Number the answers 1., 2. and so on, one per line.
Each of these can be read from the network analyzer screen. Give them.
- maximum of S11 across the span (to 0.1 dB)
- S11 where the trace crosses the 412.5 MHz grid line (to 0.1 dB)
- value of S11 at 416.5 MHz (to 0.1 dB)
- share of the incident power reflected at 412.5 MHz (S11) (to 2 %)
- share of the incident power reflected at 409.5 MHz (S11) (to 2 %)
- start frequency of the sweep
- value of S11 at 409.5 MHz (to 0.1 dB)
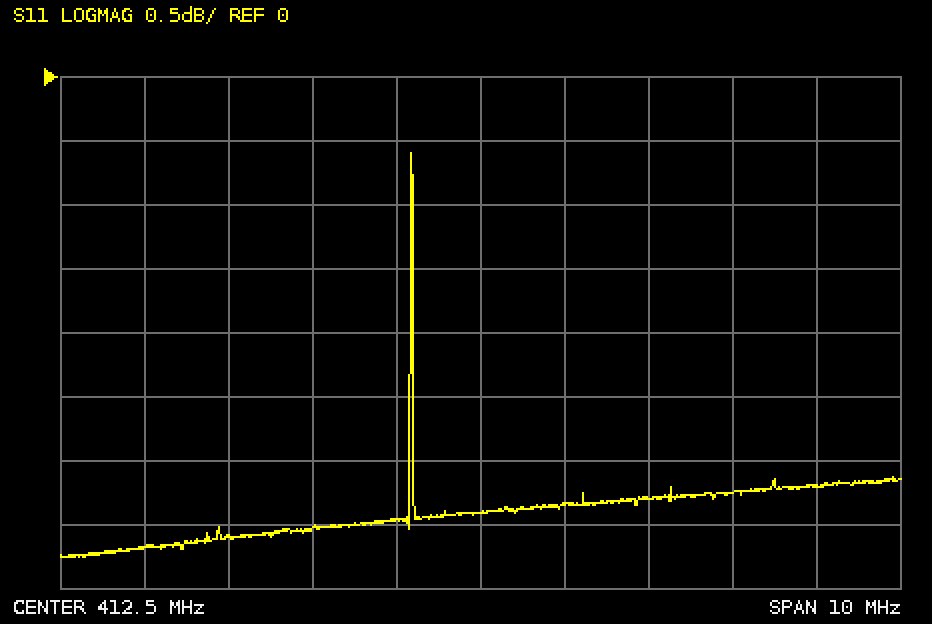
1. -0.6 dB
2. -3.4 dB
3. -3.2 dB
4. 46 %
5. 44 %
6. 407.5 MHz
7. -3.6 dB
